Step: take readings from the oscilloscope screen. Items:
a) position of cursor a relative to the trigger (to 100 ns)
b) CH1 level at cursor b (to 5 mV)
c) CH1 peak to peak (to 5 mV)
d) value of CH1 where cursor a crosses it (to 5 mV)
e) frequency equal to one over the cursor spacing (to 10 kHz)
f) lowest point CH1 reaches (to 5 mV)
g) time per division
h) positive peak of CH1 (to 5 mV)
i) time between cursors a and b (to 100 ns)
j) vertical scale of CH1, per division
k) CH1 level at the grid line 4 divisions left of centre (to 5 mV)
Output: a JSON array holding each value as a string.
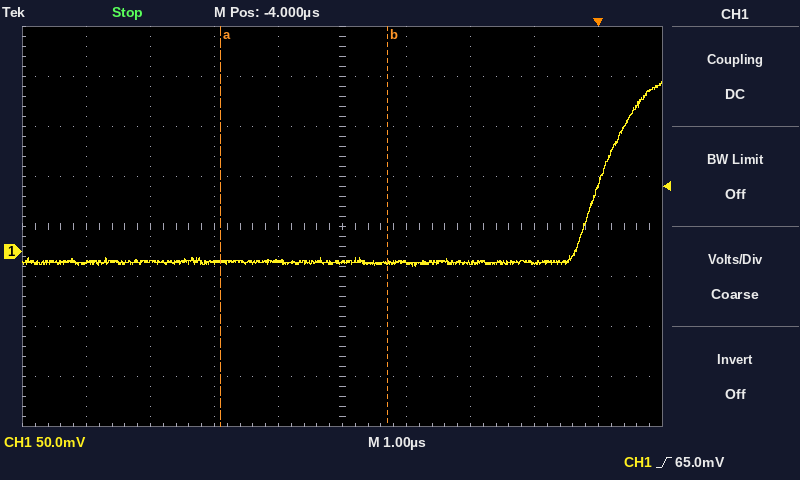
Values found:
["-5.9 µs", "-10 mV", "185 mV", "-10 mV", "380 kHz", "-15 mV", "1 µs", "170 mV", "2.6 µs", "50 mV", "-10 mV"]
